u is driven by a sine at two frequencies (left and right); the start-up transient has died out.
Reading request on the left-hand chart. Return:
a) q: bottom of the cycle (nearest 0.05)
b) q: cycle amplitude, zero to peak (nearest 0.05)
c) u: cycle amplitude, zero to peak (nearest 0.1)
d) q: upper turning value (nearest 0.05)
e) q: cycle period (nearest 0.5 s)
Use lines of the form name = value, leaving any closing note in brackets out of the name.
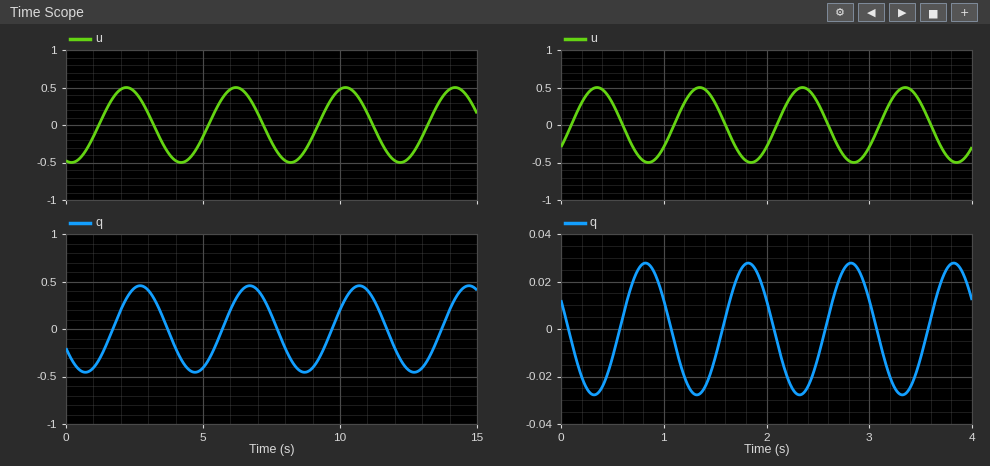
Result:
q: bottom of the cycle = -0.45
q: cycle amplitude, zero to peak = 0.45
u: cycle amplitude, zero to peak = 0.5
q: upper turning value = 0.45
q: cycle period = 4.0 s
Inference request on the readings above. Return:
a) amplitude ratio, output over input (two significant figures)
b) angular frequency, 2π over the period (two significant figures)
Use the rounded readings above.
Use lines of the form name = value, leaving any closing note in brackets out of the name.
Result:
amplitude ratio, output over input = 0.90
angular frequency, 2π over the period = 1.6 rad/s
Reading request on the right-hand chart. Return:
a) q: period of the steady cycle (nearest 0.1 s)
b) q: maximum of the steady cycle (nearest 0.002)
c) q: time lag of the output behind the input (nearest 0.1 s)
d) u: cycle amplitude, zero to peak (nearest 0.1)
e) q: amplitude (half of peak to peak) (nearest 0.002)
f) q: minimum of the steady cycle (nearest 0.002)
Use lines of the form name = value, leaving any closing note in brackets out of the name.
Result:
q: period of the steady cycle = 1.0 s
q: maximum of the steady cycle = 0.028
q: time lag of the output behind the input = 0.5 s
u: cycle amplitude, zero to peak = 0.5
q: amplitude (half of peak to peak) = 0.028
q: minimum of the steady cycle = -0.028
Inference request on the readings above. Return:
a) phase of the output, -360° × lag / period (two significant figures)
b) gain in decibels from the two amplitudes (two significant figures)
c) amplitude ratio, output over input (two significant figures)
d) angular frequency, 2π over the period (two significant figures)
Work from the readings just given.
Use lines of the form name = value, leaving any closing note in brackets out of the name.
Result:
phase of the output, -360° × lag / period = -180°
gain in decibels from the two amplitudes = -25 dB
amplitude ratio, output over input = 0.056
angular frequency, 2π over the period = 6.3 rad/s
